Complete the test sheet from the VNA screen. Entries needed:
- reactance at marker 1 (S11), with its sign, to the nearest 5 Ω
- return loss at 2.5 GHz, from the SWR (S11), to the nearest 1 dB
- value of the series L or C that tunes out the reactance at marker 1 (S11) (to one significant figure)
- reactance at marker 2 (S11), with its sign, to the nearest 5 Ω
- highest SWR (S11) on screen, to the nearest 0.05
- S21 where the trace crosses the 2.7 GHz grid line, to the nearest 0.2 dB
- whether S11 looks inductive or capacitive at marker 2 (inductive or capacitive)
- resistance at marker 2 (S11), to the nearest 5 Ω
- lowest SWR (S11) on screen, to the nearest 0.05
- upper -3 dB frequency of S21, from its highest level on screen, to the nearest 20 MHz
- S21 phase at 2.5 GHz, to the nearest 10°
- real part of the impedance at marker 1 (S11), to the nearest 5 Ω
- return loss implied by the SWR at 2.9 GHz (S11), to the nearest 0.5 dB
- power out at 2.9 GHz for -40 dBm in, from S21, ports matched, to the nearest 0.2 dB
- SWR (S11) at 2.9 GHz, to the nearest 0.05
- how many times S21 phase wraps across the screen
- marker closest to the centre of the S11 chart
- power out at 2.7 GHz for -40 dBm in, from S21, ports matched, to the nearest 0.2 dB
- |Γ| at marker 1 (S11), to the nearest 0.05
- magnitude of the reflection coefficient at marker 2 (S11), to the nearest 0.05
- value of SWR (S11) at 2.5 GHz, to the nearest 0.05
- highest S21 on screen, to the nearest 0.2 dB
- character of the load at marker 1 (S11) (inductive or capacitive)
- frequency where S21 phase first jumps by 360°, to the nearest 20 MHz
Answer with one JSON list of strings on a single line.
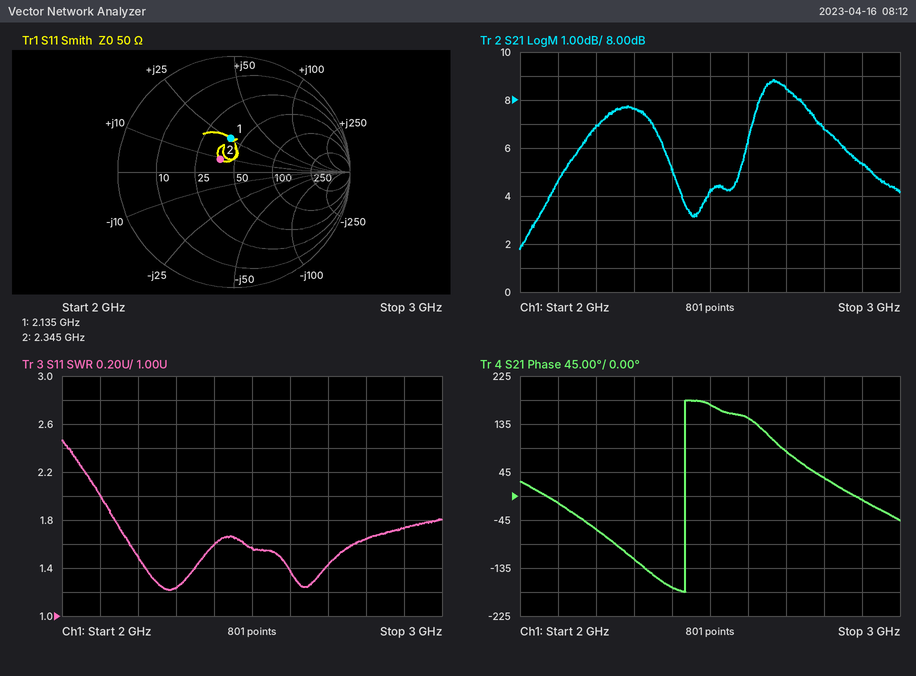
["+25 Ω", "13 dB", "3 pF", "+10 Ω", "2.45", "8.4 dB", "inductive", "40 Ω", "1.20", "2.86 GHz", "170°", "40 Ω", "11.5 dB", "-34.6 dBm", "1.75", "1", "marker 2", "-31.6 dBm", "0.30", "0.15", "1.55", "8.8 dB", "inductive", "2.44 GHz"]
